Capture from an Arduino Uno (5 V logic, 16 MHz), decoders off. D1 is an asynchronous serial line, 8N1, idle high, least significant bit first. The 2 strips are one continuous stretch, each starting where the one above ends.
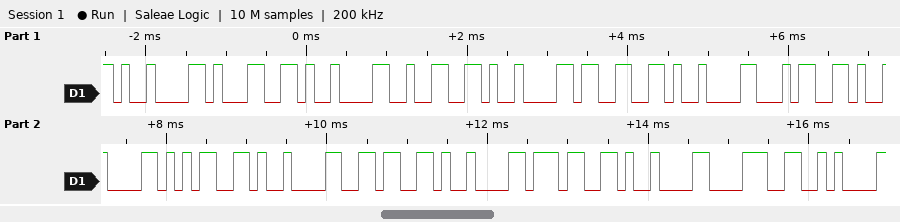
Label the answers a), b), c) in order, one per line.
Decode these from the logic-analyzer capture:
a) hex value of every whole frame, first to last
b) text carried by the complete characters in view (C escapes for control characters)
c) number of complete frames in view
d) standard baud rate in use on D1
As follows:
a) 09 31 09 32 09 33 09 34 09 35 09 36 09 37 09 38 0A
b) "\t1\t2\t3\t4\t5\t6\t7\t8\n"
c) 17
d) 9600 baud
